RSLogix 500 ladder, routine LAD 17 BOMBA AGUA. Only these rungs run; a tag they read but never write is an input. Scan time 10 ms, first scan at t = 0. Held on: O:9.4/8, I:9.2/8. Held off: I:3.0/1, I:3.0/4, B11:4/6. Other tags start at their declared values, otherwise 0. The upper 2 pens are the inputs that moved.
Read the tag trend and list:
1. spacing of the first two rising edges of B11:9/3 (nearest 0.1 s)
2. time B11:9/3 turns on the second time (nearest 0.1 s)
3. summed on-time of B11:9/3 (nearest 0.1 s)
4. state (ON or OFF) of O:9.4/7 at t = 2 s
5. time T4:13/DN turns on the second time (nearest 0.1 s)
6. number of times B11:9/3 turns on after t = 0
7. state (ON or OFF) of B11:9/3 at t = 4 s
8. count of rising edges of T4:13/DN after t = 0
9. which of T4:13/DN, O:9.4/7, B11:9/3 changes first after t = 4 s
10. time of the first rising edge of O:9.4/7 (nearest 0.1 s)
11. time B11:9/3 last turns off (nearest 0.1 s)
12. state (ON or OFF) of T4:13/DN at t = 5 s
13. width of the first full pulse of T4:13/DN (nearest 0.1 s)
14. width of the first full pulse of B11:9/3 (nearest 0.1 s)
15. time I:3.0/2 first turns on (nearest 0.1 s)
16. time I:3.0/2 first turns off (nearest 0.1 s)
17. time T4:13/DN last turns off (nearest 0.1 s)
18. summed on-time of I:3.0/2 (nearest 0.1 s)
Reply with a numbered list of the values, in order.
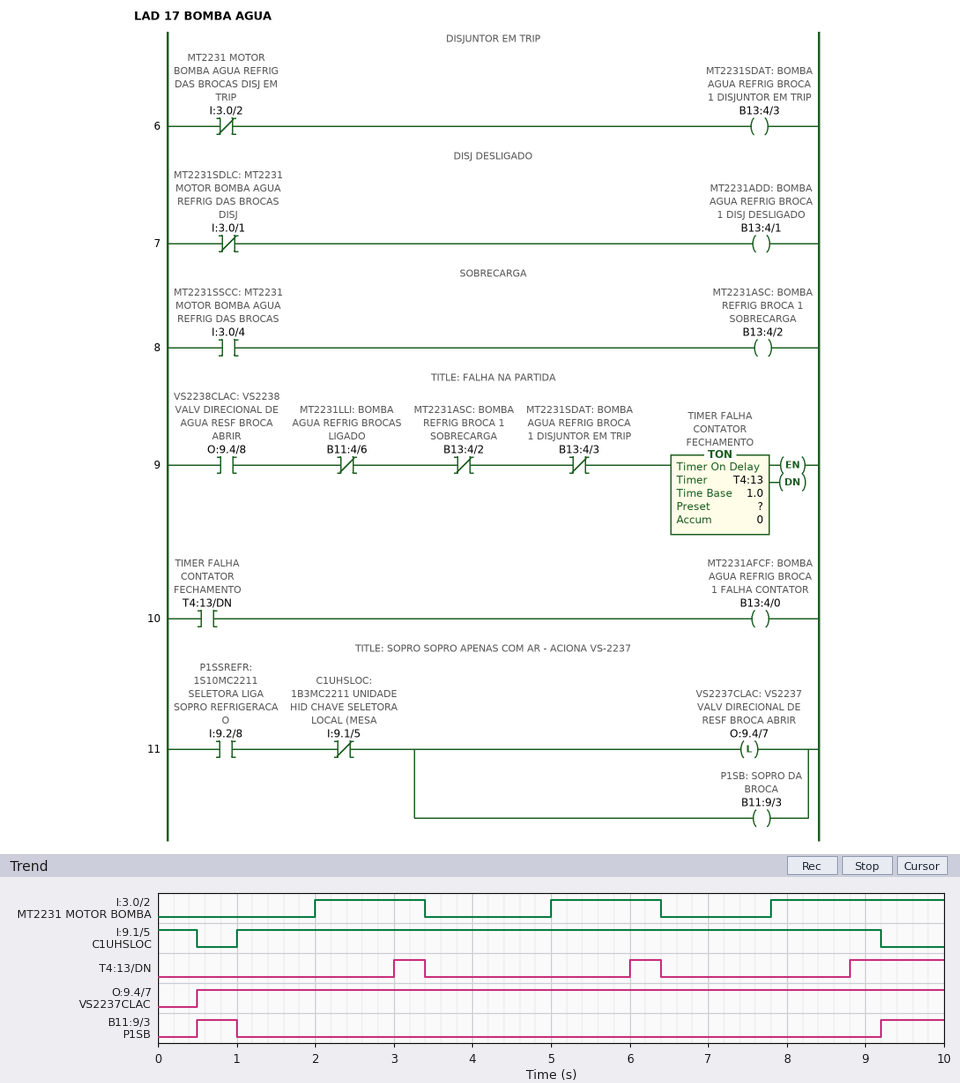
1. 8.7 s
2. 9.2 s
3. 1.3 s
4. ON
5. 6.0 s
6. 2
7. OFF
8. 3
9. T4:13/DN
10. 0.5 s
11. 1.0 s
12. OFF
13. 0.4 s
14. 0.5 s
15. 2.0 s
16. 3.4 s
17. 6.4 s
18. 5.0 s
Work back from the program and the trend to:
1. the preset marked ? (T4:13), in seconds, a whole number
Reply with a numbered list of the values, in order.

1. 1 s
